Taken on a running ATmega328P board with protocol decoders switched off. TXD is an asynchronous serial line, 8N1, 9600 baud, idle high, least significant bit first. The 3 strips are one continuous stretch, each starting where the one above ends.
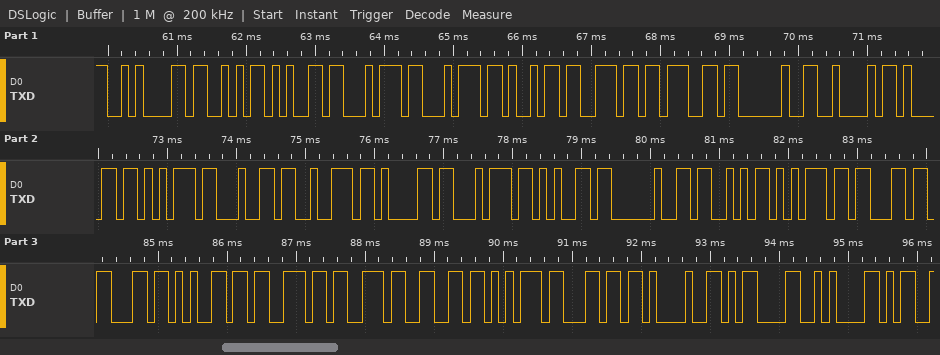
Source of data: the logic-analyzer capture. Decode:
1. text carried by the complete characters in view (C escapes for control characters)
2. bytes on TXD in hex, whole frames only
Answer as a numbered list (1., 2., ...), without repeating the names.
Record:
1. "\nSetting Baudrate Successful!\r\n"
2. 0x0A 0x53 0x65 0x74 0x74 0x69 0x6E 0x67 0x20 0x42 0x61 0x75 0x64 0x72 0x61 0x74 0x65 0x20 0x53 0x75 0x63 0x63 0x65 0x73 0x73 0x66 0x75 0x6C 0x21 0x0D 0x0A
